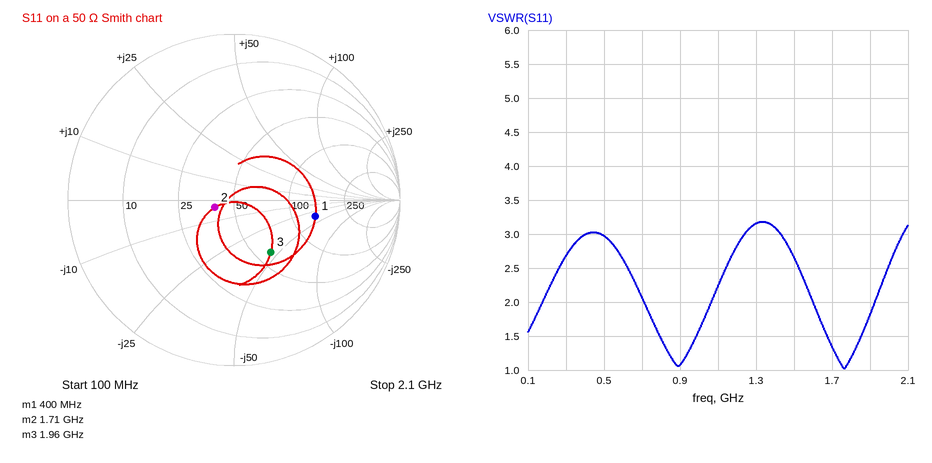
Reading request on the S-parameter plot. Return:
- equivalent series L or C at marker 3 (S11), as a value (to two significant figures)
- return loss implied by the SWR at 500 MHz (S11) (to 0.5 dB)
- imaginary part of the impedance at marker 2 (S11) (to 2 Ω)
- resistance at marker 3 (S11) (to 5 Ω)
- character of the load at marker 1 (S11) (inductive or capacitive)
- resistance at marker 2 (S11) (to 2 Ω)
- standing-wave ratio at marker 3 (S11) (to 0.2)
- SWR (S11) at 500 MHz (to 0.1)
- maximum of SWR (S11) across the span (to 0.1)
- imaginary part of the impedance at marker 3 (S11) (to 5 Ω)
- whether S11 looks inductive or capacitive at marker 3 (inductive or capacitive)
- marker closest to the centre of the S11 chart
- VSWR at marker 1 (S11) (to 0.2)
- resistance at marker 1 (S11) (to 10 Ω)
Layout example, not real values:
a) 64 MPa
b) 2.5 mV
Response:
a) 1.8 pF
b) 6.0 dB
c) -4 Ω
d) 60 Ω
e) capacitive
f) 40 Ω
g) 2.2
h) 3.0
i) 3.2
j) -45 Ω
k) capacitive
l) marker 2
m) 3.0
n) 140 Ω
